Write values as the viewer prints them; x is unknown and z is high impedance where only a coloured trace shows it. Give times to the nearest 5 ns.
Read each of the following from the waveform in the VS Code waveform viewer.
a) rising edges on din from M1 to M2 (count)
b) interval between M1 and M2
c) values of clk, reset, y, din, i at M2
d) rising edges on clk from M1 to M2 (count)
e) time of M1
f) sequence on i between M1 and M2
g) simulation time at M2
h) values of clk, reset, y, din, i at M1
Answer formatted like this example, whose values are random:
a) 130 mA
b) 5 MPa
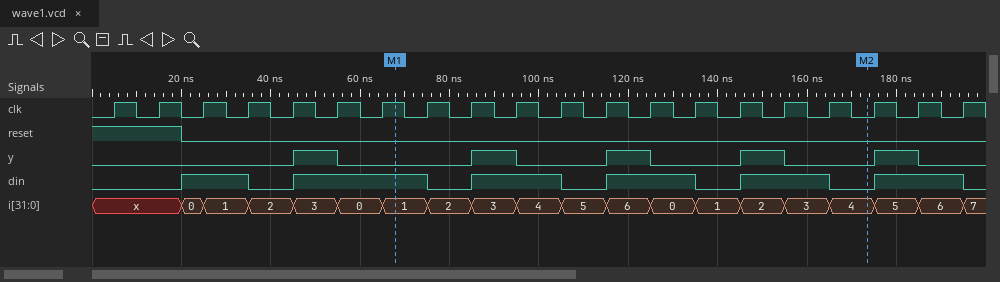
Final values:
a) 3
b) 105 ns
c) clk=0, reset=0, y=0, din=0, i=4
d) 10
e) 70 ns
f) 1, 2, 3, 4, 5, 6, 0, 1, 2, 3, 4
g) 175 ns
h) clk=1, reset=0, y=0, din=1, i=1
